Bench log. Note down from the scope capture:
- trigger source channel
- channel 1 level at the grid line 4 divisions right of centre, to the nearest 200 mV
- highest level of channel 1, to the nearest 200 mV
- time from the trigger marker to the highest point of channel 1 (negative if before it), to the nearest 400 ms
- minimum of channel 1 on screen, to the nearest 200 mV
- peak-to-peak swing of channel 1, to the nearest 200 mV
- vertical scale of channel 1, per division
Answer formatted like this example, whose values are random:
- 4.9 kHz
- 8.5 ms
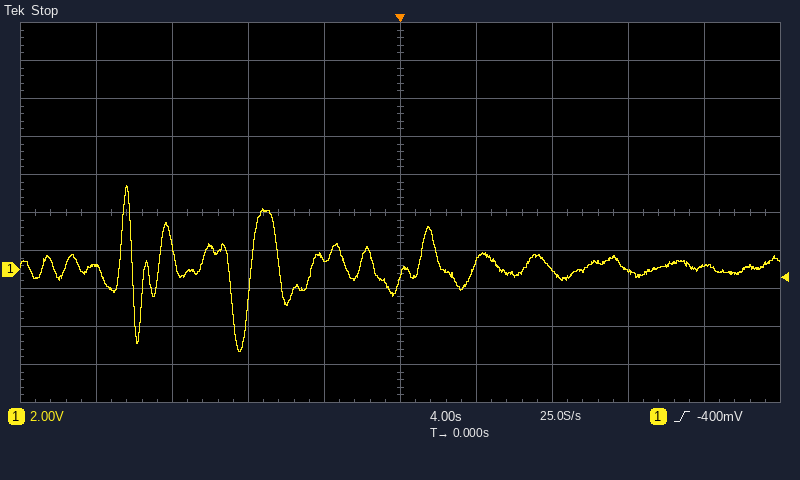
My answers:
- channel 1
- 200 mV
- 4.4 V
- -14.4 s
- -4.4 V
- 8.8 V
- 2 V
